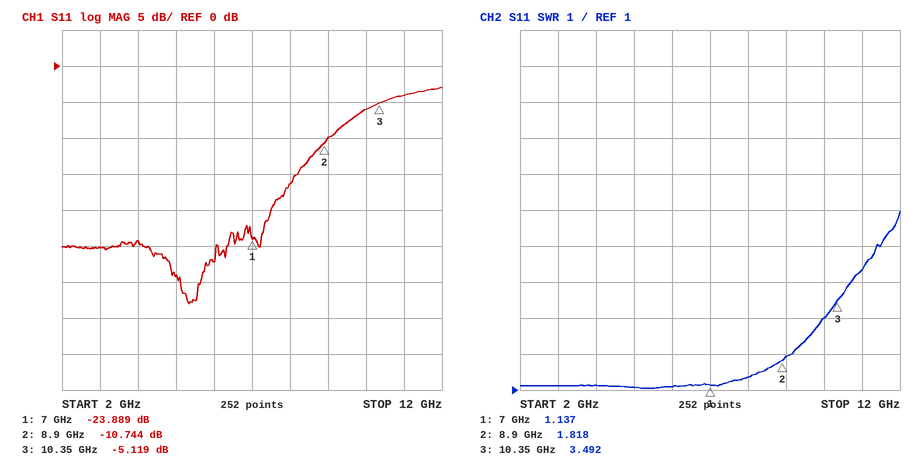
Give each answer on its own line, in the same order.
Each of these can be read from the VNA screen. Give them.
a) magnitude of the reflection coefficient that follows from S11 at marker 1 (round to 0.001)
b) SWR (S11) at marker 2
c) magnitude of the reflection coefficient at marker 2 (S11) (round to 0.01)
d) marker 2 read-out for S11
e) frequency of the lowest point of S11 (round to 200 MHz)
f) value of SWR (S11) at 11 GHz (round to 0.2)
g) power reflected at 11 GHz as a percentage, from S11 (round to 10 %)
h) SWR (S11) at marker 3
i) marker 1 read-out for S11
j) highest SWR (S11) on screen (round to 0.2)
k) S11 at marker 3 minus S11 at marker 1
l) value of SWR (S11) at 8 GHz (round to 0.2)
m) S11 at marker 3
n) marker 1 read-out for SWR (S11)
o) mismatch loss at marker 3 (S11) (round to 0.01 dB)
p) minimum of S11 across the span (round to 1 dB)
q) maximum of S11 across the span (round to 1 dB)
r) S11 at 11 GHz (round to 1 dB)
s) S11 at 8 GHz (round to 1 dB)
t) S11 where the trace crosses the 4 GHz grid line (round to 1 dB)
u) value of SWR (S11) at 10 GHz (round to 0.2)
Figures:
0.064
1.818
0.29
-10.744 dB
5.4 GHz
4.4
40 %
3.492
-23.889 dB
6.0
18.770 dB
1.4
-5.119 dB
1.137
1.60 dB
-33 dB
-3 dB
-4 dB
-16 dB
-24 dB
3.0
